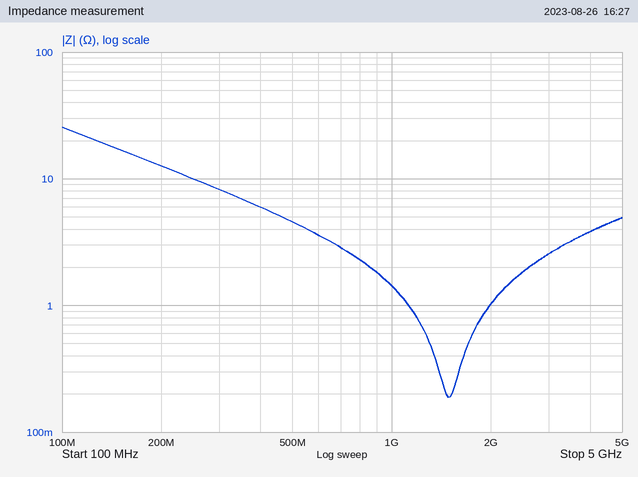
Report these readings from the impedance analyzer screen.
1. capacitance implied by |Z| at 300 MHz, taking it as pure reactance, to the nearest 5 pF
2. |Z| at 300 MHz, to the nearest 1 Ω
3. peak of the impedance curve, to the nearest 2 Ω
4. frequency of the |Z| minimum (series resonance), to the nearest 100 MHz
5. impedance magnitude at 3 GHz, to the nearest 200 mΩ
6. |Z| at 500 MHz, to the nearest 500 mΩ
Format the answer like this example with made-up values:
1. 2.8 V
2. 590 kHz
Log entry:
1. 65 pF
2. 8 Ω
3. 26 Ω
4. 1.5 GHz
5. 2.6 Ω
6. 4.5 Ω
